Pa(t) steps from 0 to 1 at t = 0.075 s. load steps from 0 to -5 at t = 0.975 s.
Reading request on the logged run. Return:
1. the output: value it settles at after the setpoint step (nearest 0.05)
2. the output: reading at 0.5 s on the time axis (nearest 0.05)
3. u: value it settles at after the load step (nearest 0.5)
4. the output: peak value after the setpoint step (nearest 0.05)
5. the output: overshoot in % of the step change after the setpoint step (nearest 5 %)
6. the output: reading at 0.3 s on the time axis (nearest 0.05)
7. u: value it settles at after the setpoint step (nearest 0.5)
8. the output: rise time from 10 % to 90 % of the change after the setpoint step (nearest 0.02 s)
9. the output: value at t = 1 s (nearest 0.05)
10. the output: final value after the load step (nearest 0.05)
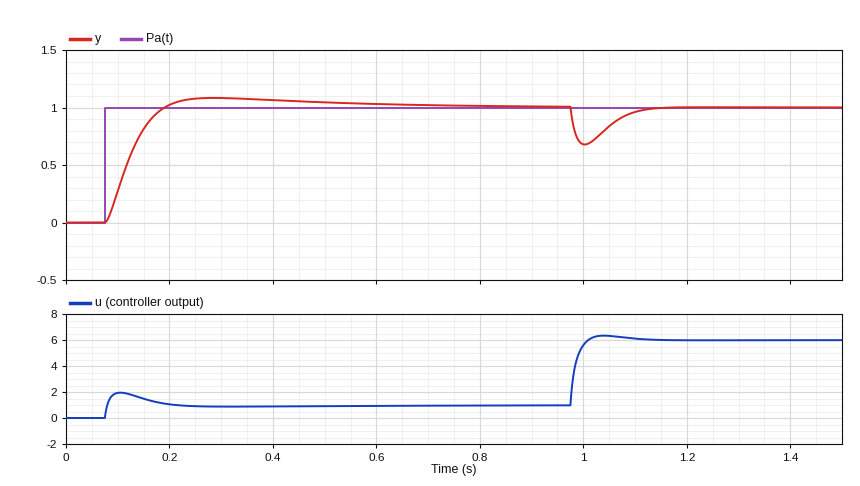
1.00
1.05
6.0
1.10
10 %
1.10
1.0
0.08 s
0.70
1.00
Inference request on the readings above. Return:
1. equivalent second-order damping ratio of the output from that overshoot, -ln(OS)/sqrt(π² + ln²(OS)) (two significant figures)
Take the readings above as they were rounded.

0.59
